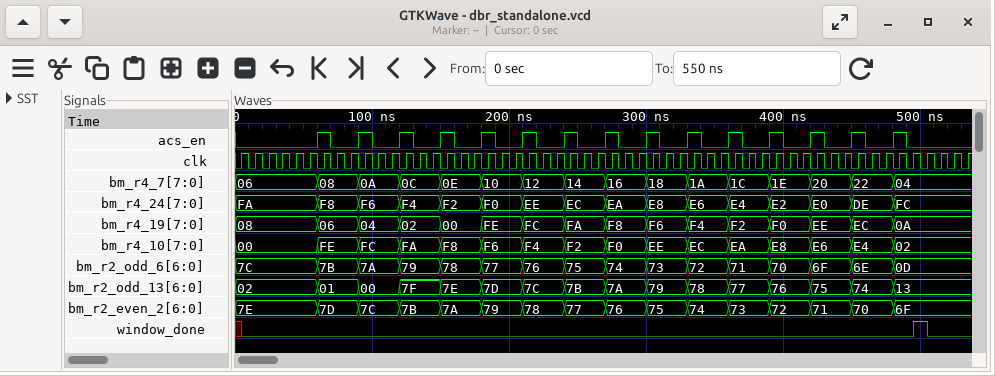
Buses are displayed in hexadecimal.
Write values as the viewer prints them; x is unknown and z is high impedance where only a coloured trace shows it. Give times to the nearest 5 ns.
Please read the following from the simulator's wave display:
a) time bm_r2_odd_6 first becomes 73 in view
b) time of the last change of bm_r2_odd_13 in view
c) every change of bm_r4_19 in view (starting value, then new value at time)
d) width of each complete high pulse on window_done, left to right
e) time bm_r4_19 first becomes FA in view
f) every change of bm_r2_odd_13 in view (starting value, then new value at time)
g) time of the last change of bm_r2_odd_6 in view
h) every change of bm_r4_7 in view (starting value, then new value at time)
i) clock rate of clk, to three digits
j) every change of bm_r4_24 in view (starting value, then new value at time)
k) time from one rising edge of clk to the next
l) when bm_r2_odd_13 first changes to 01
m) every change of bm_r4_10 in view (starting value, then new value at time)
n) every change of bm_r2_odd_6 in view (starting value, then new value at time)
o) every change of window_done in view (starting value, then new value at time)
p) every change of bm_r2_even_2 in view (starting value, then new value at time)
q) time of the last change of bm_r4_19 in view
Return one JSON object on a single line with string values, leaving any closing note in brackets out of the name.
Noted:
{"time bm_r2_odd_6 first becomes 73 in view": "300 ns", "time of the last change of bm_r2_odd_13 in view": "480 ns", "every change of bm_r4_19 in view": "08, 06 at 60 ns, 04 at 90 ns, 02 at 120 ns, 00 at 150 ns, FE at 180 ns, FC at 210 ns, FA at 240 ns, F8 at 270 ns, F6 at 300 ns, F4 at 330 ns, F2 at 360 ns, F0 at 390 ns, EE at 420 ns, EC at 450 ns, 0A at 480 ns", "width of each complete high pulse on window_done, left to right": "10 ns", "time bm_r4_19 first becomes FA in view": "240 ns", "every change of bm_r2_odd_13 in view": "02, 01 at 60 ns, 00 at 90 ns, 7F at 120 ns, 7E at 150 ns, 7D at 180 ns, 7C at 210 ns, 7B at 240 ns, 7A at 270 ns, 79 at 300 ns, 78 at 330 ns, 77 at 360 ns, 76 at 390 ns, 75 at 420 ns, 74 at 450 ns, 13 at 480 ns", "time of the last change of bm_r2_odd_6 in view": "480 ns", "every change of bm_r4_7 in view": "06, 08 at 60 ns, 0A at 90 ns, 0C at 120 ns, 0E at 150 ns, 10 at 180 ns, 12 at 210 ns, 14 at 240 ns, 16 at 270 ns, 18 at 300 ns, 1A at 330 ns, 1C at 360 ns, 1E at 390 ns, 20 at 420 ns, 22 at 450 ns, 04 at 480 ns", "clock rate of clk, to three digits": "100 MHz", "every change of bm_r4_24 in view": "FA, F8 at 60 ns, F6 at 90 ns, F4 at 120 ns, F2 at 150 ns, F0 at 180 ns, EE at 210 ns, EC at 240 ns, EA at 270 ns, E8 at 300 ns, E6 at 330 ns, E4 at 360 ns, E2 at 390 ns, E0 at 420 ns, DE at 450 ns, FC at 480 ns", "time from one rising edge of clk to the next": "10 ns", "when bm_r2_odd_13 first changes to 01": "60 ns", "every change of bm_r4_10 in view": "00, FE at 60 ns, FC at 90 ns, FA at 120 ns, F8 at 150 ns, F6 at 180 ns, F4 at 210 ns, F2 at 240 ns, F0 at 270 ns, EE at 300 ns, EC at 330 ns, EA at 360 ns, E8 at 390 ns, E6 at 420 ns, E4 at 450 ns, 02 at 480 ns", "every change of bm_r2_odd_6 in view": "7C, 7B at 60 ns, 7A at 90 ns, 79 at 120 ns, 78 at 150 ns, 77 at 180 ns, 76 at 210 ns, 75 at 240 ns, 74 at 270 ns, 73 at 300 ns, 72 at 330 ns, 71 at 360 ns, 70 at 390 ns, 6F at 420 ns, 6E at 450 ns, 0D at 480 ns", "every change of window_done in view": "x, 0 at 5 ns, 1 at 495 ns, 0 at 505 ns", "every change of bm_r2_even_2 in view": "7E, 7D at 60 ns, 7C at 90 ns, 7B at 120 ns, 7A at 150 ns, 79 at 180 ns, 78 at 210 ns, 77 at 240 ns, 76 at 270 ns, 75 at 300 ns, 74 at 330 ns, 73 at 360 ns, 72 at 390 ns, 71 at 420 ns, 70 at 450 ns, 6F at 480 ns", "time of the last change of bm_r4_19 in view": "480 ns"}
